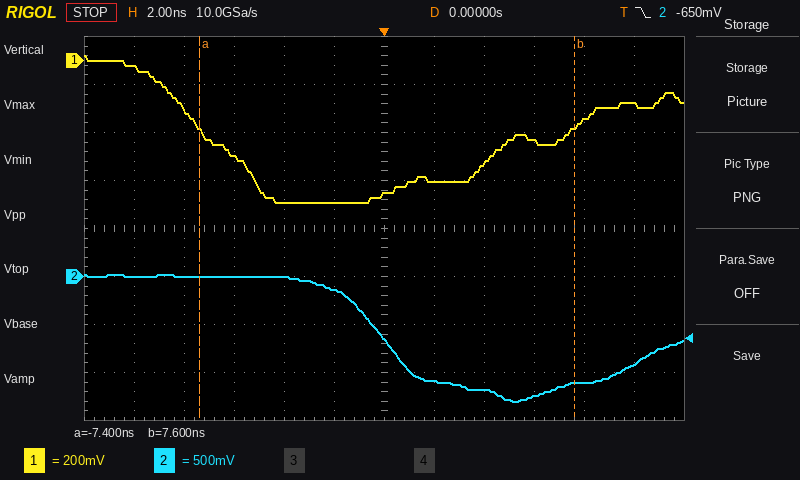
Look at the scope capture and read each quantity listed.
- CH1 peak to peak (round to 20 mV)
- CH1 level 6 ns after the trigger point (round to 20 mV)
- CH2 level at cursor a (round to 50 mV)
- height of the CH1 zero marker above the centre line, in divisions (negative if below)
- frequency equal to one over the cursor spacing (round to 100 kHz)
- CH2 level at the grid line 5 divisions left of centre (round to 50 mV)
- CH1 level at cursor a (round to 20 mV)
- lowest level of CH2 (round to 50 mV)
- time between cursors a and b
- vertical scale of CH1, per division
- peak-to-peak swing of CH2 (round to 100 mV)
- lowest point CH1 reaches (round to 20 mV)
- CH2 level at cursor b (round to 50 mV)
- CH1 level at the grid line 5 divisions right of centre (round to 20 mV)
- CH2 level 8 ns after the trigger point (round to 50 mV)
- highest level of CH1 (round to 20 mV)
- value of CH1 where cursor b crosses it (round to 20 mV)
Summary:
620 mV
-340 mV
0 mV
+3.5 div
66.7 MHz
0 mV
-280 mV
-1.30 V
15.0 ns
200 mV
1.30 V
-600 mV
-1.10 V
-180 mV
-1.10 V
20 mV
-280 mV
